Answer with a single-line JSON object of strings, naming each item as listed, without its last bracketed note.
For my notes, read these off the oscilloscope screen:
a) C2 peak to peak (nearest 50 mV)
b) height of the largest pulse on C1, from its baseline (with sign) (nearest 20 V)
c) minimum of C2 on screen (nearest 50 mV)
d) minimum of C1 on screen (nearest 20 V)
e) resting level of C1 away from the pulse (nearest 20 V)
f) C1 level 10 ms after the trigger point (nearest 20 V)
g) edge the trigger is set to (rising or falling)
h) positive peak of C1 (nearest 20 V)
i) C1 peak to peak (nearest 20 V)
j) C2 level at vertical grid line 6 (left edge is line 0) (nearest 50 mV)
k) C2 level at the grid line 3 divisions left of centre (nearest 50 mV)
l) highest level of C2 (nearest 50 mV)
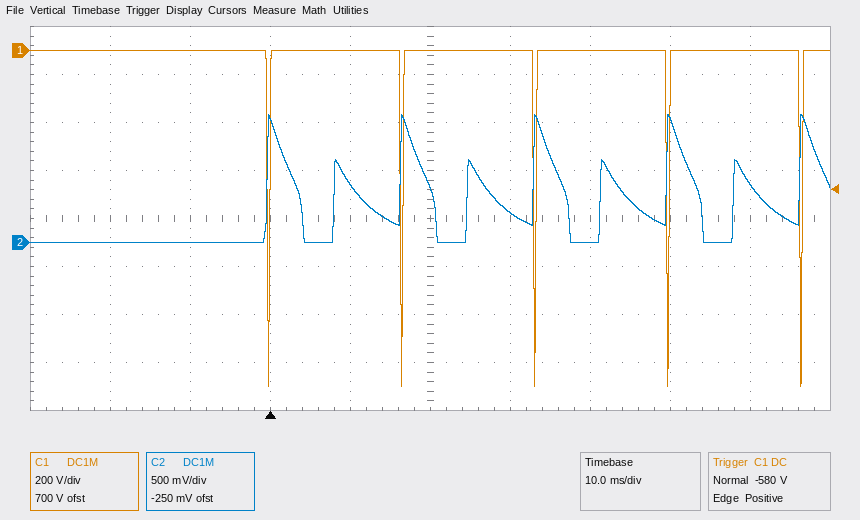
{"C2 peak to peak": "1.35 V", "height of the largest pulse on C1, from its baseline (with sign)": "-1.40 kV", "minimum of C2 on screen": "0 mV", "minimum of C1 on screen": "-1.40 kV", "resting level of C1 away from the pulse": "0 V", "C1 level 10 ms after the trigger point": "0 V", "edge the trigger is set to": "rising", "positive peak of C1": "0 V", "C1 peak to peak": "1.40 kV", "C2 level at vertical grid line 6 (left edge is line 0)": "300 mV", "C2 level at the grid line 3 divisions left of centre": "0 mV", "highest level of C2": "1.35 V"}
